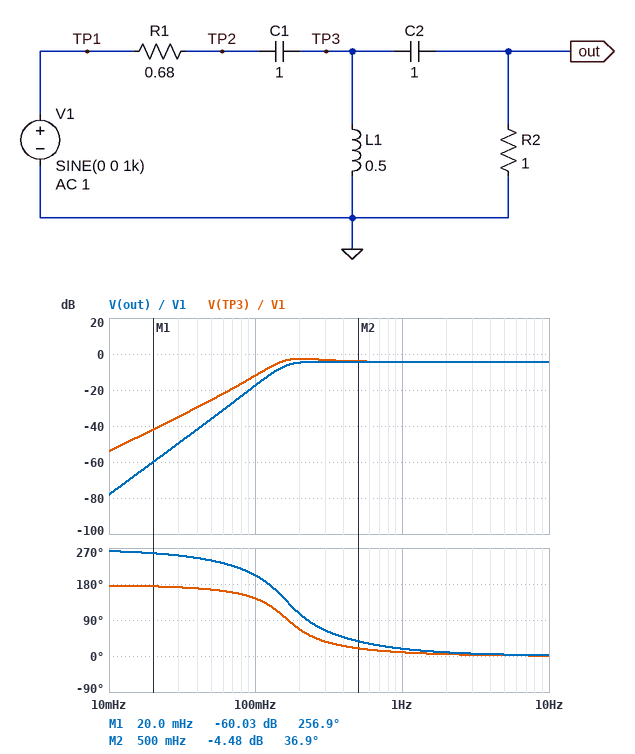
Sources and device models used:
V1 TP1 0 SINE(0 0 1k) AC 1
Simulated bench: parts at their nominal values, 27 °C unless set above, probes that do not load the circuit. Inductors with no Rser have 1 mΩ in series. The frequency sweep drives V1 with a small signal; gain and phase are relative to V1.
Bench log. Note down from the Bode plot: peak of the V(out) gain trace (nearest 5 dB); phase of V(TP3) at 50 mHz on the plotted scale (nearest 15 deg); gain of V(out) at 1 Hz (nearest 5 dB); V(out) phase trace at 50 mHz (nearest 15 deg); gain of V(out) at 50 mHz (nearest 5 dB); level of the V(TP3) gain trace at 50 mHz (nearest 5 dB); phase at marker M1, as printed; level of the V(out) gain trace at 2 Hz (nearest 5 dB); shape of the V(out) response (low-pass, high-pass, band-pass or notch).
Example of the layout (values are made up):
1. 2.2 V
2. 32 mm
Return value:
1. -5 dB
2. 165 deg
3. -5 dB
4. 240 deg
5. -35 dB
6. -25 dB
7. 256.9 deg
8. -5 dB
9. high-pass
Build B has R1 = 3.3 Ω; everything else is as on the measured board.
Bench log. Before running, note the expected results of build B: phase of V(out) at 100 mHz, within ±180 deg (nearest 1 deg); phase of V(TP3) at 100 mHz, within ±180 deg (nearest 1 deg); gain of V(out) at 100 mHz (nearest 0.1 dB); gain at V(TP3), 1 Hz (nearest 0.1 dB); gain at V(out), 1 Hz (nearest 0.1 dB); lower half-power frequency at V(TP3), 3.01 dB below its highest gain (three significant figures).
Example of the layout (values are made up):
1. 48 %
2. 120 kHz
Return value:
1. 162 deg
2. 104 deg
3. -25.3 dB
4. -12.6 dB
5. -12.7 dB
6. 153 mHz
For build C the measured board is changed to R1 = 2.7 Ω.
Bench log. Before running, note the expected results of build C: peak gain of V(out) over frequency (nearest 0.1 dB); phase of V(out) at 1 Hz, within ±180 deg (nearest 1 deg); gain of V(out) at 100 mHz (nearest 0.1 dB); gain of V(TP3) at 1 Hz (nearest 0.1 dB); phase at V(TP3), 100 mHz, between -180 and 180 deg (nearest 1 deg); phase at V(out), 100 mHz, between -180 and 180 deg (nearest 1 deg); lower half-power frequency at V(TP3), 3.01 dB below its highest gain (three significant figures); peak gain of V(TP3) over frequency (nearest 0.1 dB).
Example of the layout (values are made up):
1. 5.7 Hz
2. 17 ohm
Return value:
1. -11.4 dB
2. 18 deg
3. -23.8 dB
4. -11.3 dB
5. 108 deg
6. 166 deg
7. 149 mHz
8. -10.9 dB
